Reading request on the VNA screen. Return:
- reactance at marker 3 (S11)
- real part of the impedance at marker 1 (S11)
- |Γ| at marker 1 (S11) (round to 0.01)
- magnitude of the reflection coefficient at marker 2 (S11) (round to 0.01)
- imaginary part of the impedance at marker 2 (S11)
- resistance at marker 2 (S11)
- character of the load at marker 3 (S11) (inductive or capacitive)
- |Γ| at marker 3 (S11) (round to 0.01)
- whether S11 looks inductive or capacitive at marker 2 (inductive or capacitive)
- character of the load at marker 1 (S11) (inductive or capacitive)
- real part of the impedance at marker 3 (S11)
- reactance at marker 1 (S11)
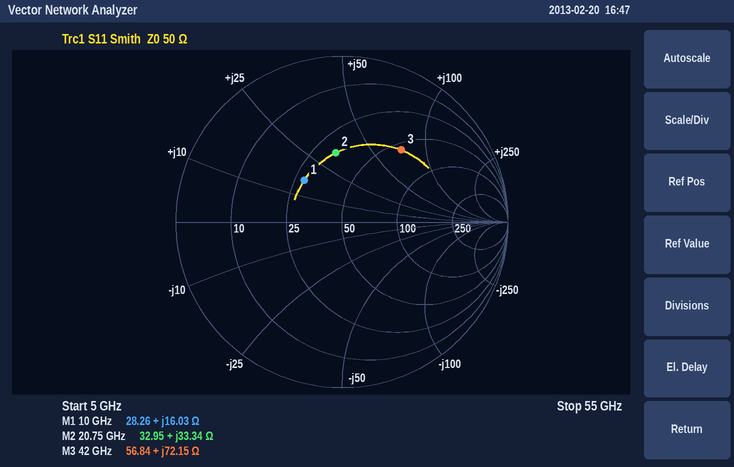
+72.15 Ω
28.26 Ω
0.34
0.42
+33.34 Ω
32.95 Ω
inductive
0.56
inductive
inductive
56.84 Ω
+16.03 Ω
